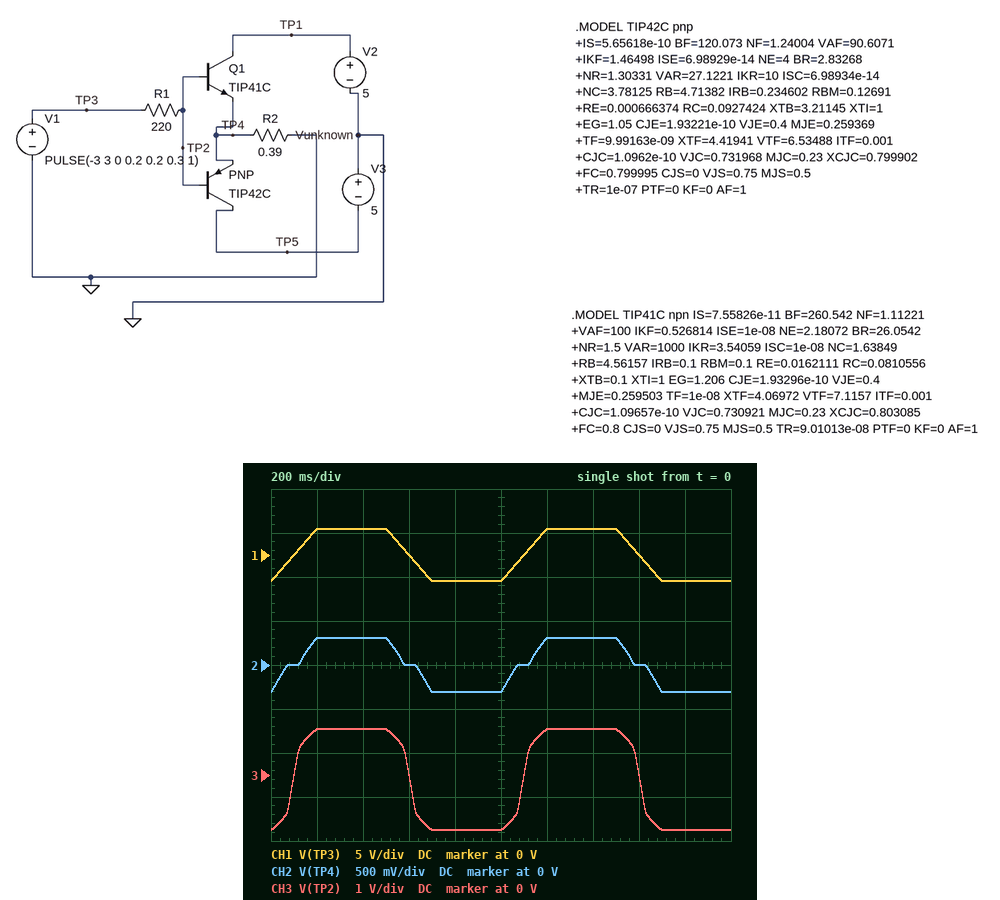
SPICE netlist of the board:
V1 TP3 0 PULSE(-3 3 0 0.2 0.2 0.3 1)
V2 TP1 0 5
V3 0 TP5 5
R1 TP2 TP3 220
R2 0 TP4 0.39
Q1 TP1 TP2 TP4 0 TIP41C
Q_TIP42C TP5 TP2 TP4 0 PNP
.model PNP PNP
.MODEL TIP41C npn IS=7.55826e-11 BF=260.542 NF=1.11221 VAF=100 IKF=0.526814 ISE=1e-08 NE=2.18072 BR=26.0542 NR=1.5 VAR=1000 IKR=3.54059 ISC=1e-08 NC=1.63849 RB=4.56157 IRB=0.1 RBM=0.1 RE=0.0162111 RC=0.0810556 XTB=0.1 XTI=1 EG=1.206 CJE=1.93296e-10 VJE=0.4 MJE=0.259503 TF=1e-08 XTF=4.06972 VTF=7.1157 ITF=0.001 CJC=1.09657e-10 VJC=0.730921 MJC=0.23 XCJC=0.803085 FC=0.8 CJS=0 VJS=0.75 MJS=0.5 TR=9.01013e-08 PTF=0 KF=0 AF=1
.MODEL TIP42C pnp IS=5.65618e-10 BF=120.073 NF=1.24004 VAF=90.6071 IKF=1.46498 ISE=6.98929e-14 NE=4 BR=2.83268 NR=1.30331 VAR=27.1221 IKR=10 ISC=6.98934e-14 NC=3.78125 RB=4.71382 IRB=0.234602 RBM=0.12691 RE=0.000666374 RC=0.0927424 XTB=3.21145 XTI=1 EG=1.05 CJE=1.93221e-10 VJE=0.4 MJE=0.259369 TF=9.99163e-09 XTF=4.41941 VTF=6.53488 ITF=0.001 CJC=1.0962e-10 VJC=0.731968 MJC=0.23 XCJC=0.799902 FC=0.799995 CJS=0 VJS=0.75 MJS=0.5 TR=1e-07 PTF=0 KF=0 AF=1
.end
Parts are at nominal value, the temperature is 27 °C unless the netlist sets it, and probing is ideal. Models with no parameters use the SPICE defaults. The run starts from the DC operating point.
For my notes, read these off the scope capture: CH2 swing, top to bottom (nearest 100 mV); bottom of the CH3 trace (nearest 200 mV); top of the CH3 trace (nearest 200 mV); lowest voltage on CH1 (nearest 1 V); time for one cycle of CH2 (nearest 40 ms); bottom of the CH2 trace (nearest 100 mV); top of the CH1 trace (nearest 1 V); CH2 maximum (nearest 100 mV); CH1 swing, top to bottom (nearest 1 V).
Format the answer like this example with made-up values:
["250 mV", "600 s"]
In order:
["600 mV", "-1.2 V", "1.0 V", "-3 V", "1.00 s", "-300 mV", "3 V", "300 mV", "6 V"]
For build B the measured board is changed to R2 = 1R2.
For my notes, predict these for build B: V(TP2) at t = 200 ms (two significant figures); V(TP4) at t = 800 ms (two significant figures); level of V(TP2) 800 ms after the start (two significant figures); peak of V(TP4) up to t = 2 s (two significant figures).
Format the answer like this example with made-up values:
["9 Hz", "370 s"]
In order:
["1.5 V", "-730 mV", "-1.7 V", "780 mV"]
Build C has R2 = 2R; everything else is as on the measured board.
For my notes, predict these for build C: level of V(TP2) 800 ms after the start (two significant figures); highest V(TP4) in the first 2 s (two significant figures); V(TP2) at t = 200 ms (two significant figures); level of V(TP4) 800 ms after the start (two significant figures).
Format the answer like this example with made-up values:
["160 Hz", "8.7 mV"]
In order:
["-1.9 V", "1.1 V", "1.8 V", "-990 mV"]
